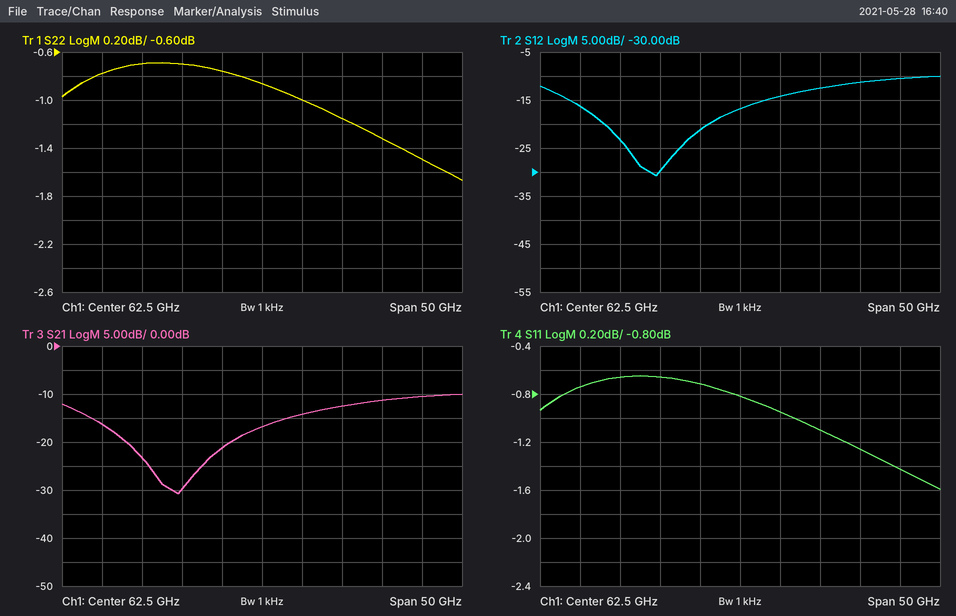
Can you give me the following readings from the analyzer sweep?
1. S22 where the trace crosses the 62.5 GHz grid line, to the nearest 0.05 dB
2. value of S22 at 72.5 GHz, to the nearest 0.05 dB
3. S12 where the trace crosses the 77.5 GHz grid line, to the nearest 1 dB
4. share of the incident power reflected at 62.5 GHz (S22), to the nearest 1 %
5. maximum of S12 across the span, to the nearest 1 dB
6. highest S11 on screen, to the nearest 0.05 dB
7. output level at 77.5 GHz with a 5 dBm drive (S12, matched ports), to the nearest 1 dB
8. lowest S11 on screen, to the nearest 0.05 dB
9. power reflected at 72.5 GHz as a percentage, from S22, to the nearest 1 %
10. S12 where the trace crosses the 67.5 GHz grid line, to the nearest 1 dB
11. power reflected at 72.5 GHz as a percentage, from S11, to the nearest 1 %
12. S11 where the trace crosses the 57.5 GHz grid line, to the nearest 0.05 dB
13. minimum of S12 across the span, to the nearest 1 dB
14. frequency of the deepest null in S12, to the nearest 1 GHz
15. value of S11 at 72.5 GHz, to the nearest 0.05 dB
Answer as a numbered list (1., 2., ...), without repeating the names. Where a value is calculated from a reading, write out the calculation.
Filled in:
1. -0.85 dB
2. -1.15 dB
3. -11 dB
4. 10^(-0.85/10) ≈ 82 %
5. -10 dB
6. -0.65 dB
7. 5 dBm + (-11 dB) = -6 dBm
8. -1.60 dB
9. 10^(-1.15/10) ≈ 77 %
10. -14 dB
11. 10^(-1.1/10) ≈ 78 %
12. -0.70 dB
13. -31 dB
14. 52 GHz
15. -1.10 dB
